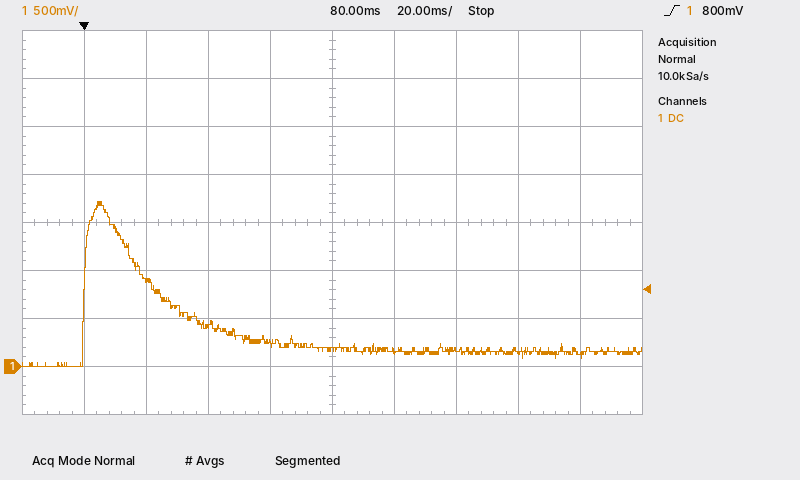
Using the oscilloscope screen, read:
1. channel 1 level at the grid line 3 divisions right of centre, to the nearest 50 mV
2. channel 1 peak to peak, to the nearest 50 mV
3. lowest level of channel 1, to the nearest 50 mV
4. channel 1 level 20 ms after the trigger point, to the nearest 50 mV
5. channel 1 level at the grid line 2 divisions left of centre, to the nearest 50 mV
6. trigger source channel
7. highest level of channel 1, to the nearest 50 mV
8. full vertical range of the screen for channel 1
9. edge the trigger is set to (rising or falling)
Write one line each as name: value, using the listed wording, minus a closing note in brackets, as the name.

channel 1 level at the grid line 3 divisions right of centre, to the nearest 50 mV: 150 mV
channel 1 peak to peak, to the nearest 50 mV: 1.70 V
lowest level of channel 1, to the nearest 50 mV: 0 mV
channel 1 level 20 ms after the trigger point, to the nearest 50 mV: 900 mV
channel 1 level at the grid line 2 divisions left of centre, to the nearest 50 mV: 450 mV
trigger source channel: channel 1
highest level of channel 1, to the nearest 50 mV: 1.70 V
full vertical range of the screen for channel 1: 4 V
edge the trigger is set to: rising
